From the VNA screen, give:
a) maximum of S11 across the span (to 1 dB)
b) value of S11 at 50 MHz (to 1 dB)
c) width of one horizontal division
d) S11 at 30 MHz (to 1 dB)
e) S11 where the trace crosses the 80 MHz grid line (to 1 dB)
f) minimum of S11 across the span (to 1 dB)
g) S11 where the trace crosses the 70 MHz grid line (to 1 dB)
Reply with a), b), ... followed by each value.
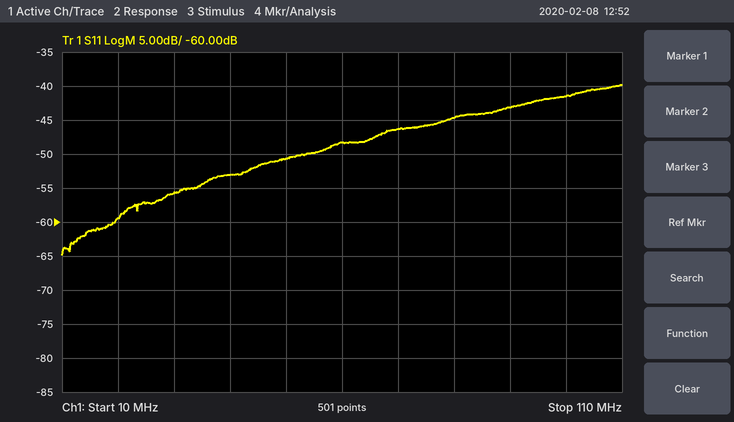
a) -40 dB
b) -51 dB
c) 10 MHz
d) -56 dB
e) -45 dB
f) -65 dB
g) -46 dB
